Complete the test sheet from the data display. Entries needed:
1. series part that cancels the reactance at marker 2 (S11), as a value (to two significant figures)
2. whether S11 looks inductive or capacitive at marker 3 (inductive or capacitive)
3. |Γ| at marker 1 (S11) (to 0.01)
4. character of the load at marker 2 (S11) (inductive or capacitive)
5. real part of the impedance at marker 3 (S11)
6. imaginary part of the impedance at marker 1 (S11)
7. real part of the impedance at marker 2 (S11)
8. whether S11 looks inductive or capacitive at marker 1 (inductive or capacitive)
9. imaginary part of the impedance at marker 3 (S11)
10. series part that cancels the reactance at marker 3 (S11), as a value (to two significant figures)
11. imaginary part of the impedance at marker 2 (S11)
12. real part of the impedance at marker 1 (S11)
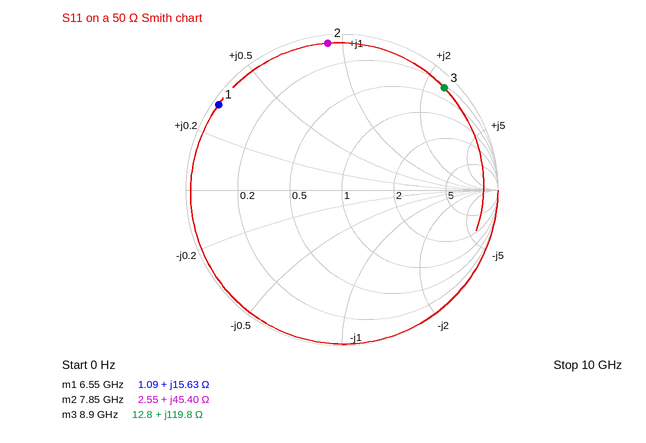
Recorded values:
450 fF
inductive
0.96
inductive
12.8 Ω
+15.63 Ω
2.55 Ω
inductive
+119.8 Ω
150 fF
+45.40 Ω
1.09 Ω
